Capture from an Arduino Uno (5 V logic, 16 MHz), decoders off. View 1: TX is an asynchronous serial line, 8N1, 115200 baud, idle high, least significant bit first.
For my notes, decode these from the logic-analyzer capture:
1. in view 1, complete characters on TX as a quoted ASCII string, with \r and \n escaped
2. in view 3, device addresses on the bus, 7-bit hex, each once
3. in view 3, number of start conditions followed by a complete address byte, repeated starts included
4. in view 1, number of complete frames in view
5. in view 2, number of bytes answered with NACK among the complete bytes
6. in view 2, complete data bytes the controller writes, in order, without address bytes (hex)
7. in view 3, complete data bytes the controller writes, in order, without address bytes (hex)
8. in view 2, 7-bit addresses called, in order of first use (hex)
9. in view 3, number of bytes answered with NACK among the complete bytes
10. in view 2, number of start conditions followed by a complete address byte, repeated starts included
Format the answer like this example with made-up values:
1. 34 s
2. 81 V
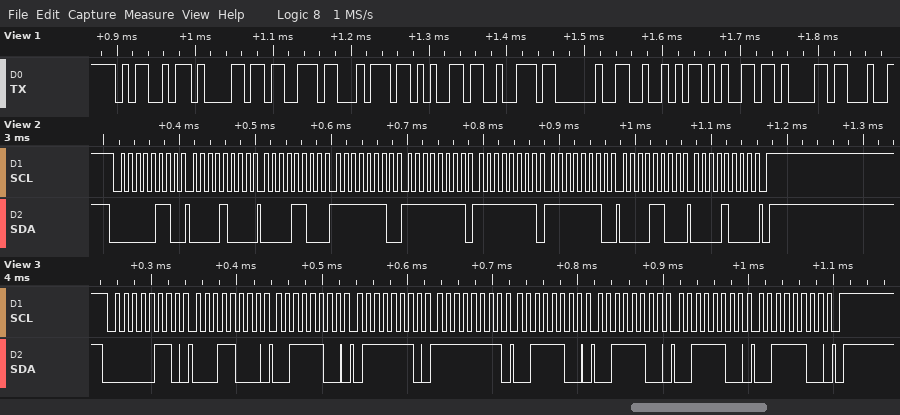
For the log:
1. "Master Rea"
2. 0x03
3. 1
4. 10
5. 0
6. 08 0C FE FF FF FE 0C 08
7. 18 3C 7E FF 3C 3C 3C 3C
8. 0x03
9. 0
10. 1
